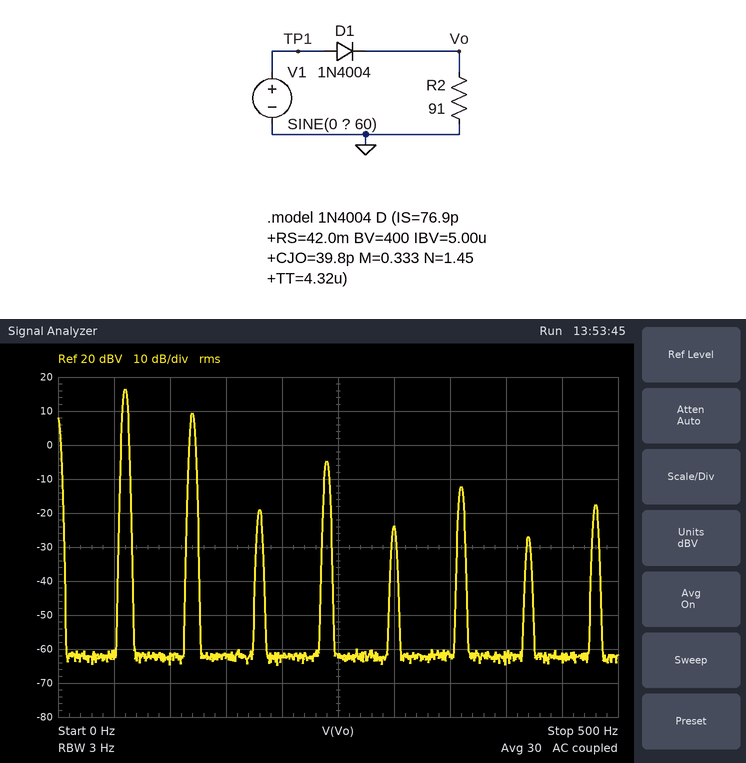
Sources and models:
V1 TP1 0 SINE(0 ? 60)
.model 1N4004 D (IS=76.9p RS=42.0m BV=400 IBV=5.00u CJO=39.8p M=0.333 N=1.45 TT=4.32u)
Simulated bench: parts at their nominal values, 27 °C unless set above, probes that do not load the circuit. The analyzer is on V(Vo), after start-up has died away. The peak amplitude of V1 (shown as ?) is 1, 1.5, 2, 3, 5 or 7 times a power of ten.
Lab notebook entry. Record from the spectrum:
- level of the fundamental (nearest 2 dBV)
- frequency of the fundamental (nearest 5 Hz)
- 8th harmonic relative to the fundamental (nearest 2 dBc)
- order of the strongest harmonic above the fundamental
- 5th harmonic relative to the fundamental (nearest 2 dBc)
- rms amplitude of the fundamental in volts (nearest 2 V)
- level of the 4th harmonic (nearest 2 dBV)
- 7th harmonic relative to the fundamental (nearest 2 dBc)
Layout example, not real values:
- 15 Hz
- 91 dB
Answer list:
- 16 dBV
- 60 Hz
- -34 dBc
- 2
- -40 dBc
- 6 V
- -4 dBV
- -44 dBc
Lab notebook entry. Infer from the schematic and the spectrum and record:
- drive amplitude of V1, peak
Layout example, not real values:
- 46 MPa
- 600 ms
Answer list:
- 20 V
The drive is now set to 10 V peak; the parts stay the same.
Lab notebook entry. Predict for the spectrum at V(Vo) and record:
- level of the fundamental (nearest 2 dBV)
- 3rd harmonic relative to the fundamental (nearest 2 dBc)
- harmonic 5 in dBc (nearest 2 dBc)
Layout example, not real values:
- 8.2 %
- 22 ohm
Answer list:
- 10 dBV
- -30 dBc
- -34 dBc
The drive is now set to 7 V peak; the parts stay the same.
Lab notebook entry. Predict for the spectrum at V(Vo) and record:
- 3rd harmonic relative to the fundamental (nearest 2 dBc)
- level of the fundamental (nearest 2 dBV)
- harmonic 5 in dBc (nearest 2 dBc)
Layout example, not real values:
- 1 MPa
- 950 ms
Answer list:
- -26 dBc
- 6 dBV
- -32 dBc
